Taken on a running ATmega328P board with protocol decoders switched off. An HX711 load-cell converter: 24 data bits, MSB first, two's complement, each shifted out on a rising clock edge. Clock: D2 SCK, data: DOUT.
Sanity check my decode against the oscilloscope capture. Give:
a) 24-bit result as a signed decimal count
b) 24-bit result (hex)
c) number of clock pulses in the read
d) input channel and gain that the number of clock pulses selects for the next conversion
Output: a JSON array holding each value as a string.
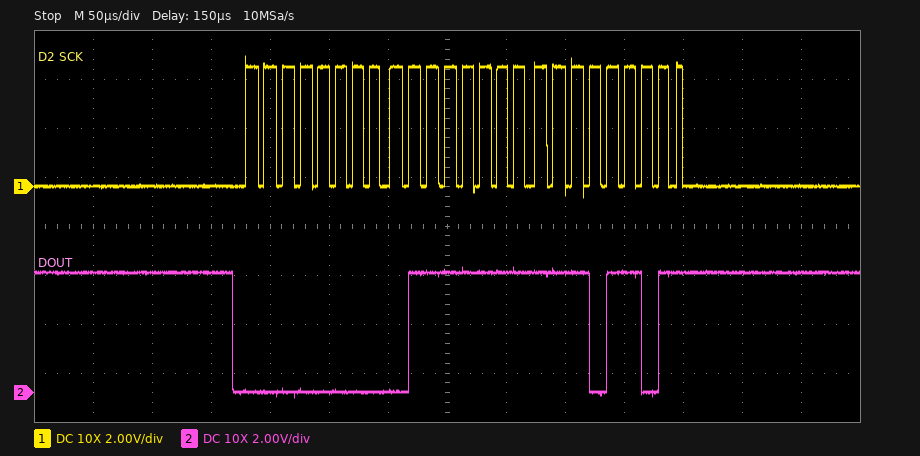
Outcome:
["32749", "0x007FED", "25", "channel A, gain 128"]
